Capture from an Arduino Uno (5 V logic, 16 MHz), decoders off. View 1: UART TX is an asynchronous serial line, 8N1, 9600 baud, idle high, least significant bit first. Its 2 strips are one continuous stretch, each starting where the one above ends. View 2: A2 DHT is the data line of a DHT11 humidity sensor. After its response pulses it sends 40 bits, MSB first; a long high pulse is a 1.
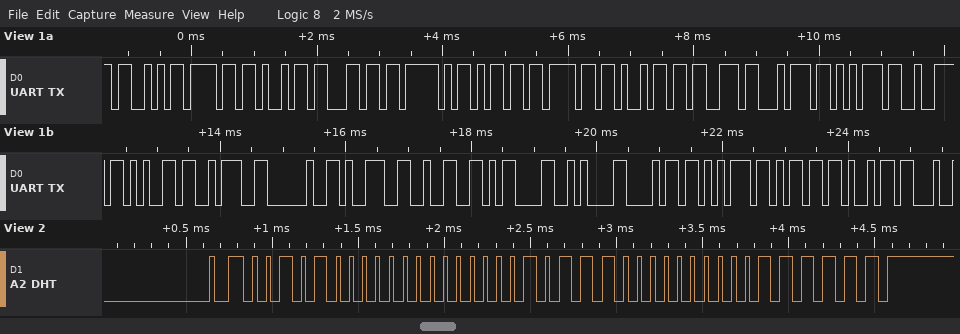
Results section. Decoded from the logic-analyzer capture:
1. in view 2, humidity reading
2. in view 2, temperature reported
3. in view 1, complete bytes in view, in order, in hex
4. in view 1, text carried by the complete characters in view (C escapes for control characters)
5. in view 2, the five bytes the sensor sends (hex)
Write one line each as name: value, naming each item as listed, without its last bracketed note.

in view 2, humidity reading: 40 %
in view 2, temperature reported: 23.0 °C
in view 1, complete bytes in view, in order, in hex: 53 6F 69 6C 5F 6D 6F 69 73 74 75 72 65 3A 20 39 32 0D 0A 68 75 6D 69
in view 1, text carried by the complete characters in view: "Soil_moisture: 92\r\nhumi"
in view 2, the five bytes the sensor sends: 28 00 17 00 3F
